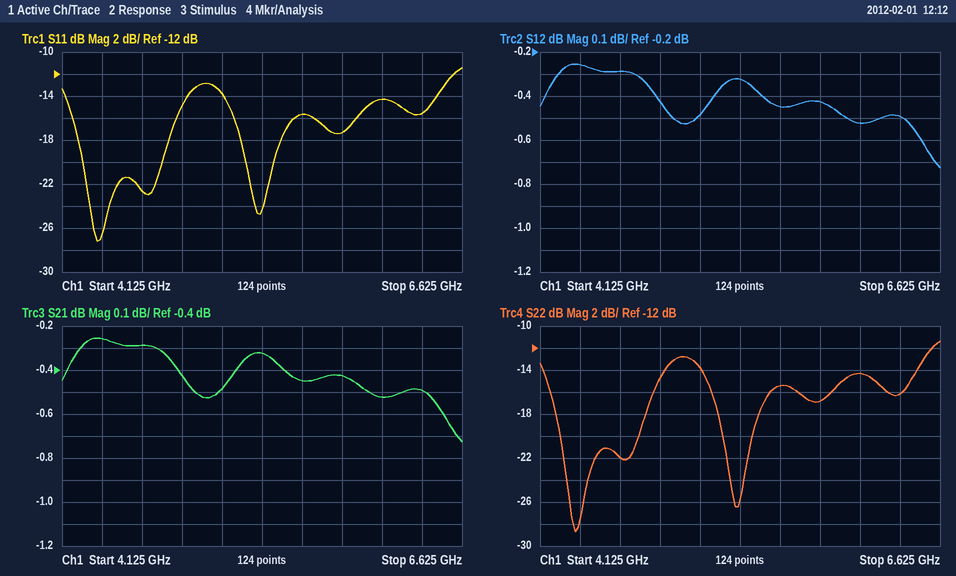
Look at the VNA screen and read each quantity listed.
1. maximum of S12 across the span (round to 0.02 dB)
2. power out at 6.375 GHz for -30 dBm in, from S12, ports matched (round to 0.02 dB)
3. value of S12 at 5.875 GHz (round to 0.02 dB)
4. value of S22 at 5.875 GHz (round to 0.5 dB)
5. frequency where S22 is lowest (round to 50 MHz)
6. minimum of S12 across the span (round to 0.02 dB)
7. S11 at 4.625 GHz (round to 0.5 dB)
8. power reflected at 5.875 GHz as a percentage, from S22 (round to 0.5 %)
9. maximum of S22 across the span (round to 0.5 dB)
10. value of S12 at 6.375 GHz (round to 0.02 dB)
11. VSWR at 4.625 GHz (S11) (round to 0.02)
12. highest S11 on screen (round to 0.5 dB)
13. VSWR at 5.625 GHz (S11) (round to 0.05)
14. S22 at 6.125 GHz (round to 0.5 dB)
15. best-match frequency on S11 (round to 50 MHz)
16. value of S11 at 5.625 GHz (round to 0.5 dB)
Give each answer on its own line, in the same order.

-0.26 dB
-30.50 dBm
-0.42 dB
-17.0 dB
4.35 GHz
-0.72 dB
-22.5 dB
2.0 %
-11.5 dB
-0.50 dB
1.16
-11.5 dB
1.40
-14.5 dB
4.35 GHz
-15.5 dB
